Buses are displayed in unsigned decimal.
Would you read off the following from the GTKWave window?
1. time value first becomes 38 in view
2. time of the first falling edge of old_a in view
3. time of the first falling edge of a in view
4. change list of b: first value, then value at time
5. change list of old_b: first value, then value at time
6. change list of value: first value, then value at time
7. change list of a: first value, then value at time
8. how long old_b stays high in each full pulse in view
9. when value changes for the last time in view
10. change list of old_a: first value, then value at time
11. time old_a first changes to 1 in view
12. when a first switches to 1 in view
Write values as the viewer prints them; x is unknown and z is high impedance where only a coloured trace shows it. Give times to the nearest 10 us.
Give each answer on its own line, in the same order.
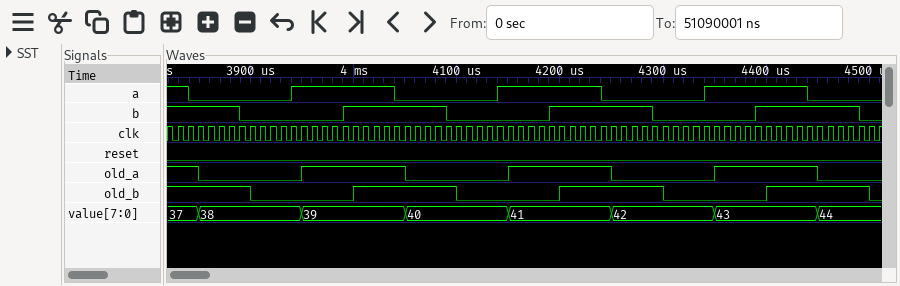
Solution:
3850 us
3850 us
3840 us
1, 0 at 3890 us, 1 at 3990 us, 0 at 4090 us, 1 at 4190 us, 0 at 4290 us, 1 at 4390 us, 0 at 4490 us
1, 0 at 3900 us, 1 at 4000 us, 0 at 4100 us, 1 at 4200 us, 0 at 4300 us, 1 at 4400 us, 0 at 4500 us
37, 38 at 3850 us, 39 at 3950 us, 40 at 4050 us, 41 at 4150 us, 42 at 4250 us, 43 at 4350 us, 44 at 4450 us
1, 0 at 3840 us, 1 at 3940 us, 0 at 4040 us, 1 at 4140 us, 0 at 4240 us, 1 at 4340 us, 0 at 4440 us
100 us, 100 us, 100 us
4450 us
1, 0 at 3850 us, 1 at 3950 us, 0 at 4050 us, 1 at 4150 us, 0 at 4250 us, 1 at 4350 us, 0 at 4450 us
3950 us
3940 us
